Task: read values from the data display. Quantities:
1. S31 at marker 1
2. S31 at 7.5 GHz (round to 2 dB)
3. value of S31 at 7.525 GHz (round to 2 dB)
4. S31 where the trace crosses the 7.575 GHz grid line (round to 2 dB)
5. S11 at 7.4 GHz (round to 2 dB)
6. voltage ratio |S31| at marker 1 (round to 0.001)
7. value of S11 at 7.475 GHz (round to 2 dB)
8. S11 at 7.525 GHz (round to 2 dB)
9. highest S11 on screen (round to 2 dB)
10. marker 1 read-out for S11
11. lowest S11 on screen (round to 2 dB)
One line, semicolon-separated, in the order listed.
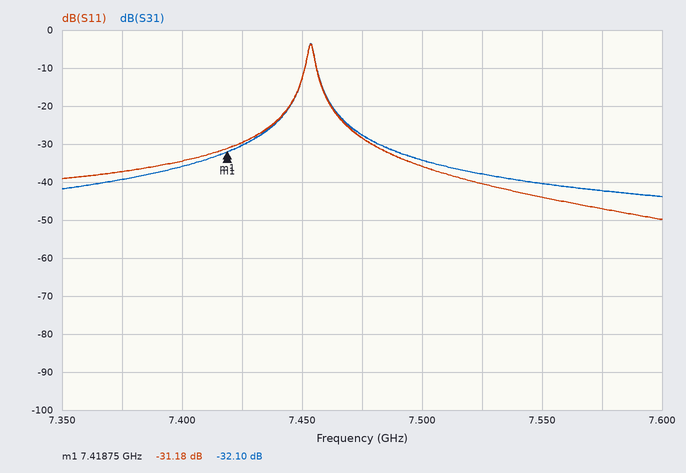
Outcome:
-32.10 dB; -34 dB; -38 dB; -42 dB; -34 dB; 0.025; -28 dB; -40 dB; -4 dB; -31.18 dB; -50 dB
